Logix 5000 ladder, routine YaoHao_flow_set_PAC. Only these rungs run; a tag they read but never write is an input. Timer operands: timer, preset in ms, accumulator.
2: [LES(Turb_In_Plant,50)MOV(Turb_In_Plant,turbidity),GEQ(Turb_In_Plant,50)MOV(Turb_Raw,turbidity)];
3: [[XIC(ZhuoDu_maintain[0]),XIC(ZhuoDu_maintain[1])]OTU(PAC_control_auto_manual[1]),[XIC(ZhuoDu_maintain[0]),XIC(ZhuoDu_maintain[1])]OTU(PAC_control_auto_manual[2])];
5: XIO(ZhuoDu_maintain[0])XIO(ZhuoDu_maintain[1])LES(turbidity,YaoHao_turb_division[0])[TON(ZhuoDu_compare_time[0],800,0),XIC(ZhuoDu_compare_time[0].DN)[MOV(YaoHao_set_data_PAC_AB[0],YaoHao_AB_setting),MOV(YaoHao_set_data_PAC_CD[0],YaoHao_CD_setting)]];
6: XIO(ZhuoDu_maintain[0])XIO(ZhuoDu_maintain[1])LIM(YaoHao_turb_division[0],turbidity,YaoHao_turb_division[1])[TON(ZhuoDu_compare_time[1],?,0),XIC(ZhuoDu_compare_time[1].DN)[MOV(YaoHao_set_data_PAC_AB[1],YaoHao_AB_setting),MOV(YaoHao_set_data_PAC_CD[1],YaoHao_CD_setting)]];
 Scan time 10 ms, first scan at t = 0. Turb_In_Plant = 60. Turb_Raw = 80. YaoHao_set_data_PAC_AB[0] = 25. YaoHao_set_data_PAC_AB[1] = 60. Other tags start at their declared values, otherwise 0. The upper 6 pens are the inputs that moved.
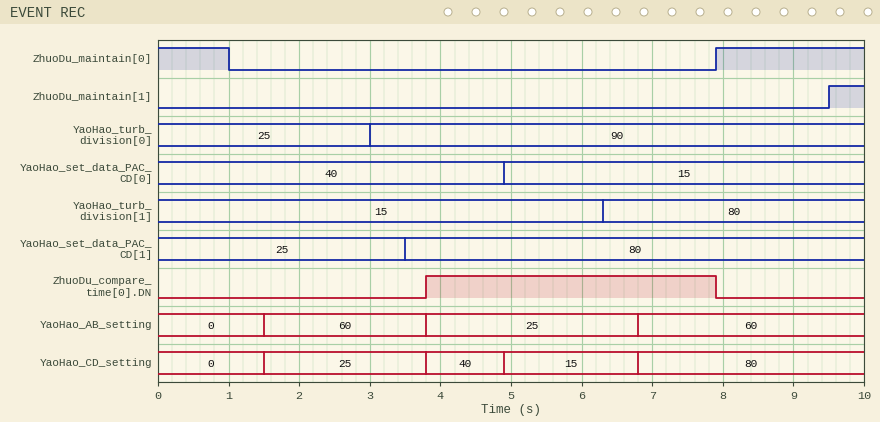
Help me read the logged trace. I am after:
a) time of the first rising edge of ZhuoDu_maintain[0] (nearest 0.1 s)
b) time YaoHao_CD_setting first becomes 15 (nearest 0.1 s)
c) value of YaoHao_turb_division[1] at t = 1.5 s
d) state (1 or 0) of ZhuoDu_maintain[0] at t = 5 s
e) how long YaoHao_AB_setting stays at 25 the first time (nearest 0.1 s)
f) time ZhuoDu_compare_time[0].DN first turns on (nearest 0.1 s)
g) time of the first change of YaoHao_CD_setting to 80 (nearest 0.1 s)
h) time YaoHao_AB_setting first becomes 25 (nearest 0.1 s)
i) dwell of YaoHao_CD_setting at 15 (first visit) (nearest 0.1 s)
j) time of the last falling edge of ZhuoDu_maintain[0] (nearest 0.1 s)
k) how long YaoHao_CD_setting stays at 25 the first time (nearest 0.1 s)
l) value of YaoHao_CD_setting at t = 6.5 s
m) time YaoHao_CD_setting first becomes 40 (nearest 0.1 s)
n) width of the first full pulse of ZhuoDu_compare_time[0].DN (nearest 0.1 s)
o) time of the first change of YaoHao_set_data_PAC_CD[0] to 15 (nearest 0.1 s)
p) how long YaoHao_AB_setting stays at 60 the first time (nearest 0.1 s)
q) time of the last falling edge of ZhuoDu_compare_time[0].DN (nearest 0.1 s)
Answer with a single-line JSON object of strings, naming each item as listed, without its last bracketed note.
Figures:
{"time of the first rising edge of ZhuoDu_maintain[0]": "7.9 s", "time YaoHao_CD_setting first becomes 15": "4.9 s", "value of YaoHao_turb_division[1] at t = 1.5 s": "15", "state (1 or 0) of ZhuoDu_maintain[0] at t = 5 s": "0", "how long YaoHao_AB_setting stays at 25 the first time": "3.0 s", "time ZhuoDu_compare_time[0].DN first turns on": "3.8 s", "time of the first change of YaoHao_CD_setting to 80": "6.8 s", "time YaoHao_AB_setting first becomes 25": "3.8 s", "dwell of YaoHao_CD_setting at 15 (first visit)": "1.9 s", "time of the last falling edge of ZhuoDu_maintain[0]": "1.0 s", "how long YaoHao_CD_setting stays at 25 the first time": "2.3 s", "value of YaoHao_CD_setting at t = 6.5 s": "15", "time YaoHao_CD_setting first becomes 40": "3.8 s", "width of the first full pulse of ZhuoDu_compare_time[0].DN": "4.1 s", "time of the first change of YaoHao_set_data_PAC_CD[0] to 15": "4.9 s", "how long YaoHao_AB_setting stays at 60 the first time": "2.3 s", "time of the last falling edge of ZhuoDu_compare_time[0].DN": "7.9 s"}
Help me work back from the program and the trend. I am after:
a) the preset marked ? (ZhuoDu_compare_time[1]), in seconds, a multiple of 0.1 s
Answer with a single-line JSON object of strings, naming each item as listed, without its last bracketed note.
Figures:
{"the preset marked ? (ZhuoDu_compare_time[1]), in seconds, a multiple of 0.1 s": "0.5 s"}
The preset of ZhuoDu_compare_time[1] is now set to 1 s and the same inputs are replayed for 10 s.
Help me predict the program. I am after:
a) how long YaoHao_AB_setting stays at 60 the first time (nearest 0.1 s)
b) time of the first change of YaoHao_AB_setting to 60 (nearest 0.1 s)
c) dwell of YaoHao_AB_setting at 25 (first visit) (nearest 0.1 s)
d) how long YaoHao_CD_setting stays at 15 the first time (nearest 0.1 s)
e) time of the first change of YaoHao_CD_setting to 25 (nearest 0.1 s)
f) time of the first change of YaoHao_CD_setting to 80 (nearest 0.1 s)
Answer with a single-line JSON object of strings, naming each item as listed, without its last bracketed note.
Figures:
{"how long YaoHao_AB_setting stays at 60 the first time": "1.8 s", "time of the first change of YaoHao_AB_setting to 60": "2.0 s", "dwell of YaoHao_AB_setting at 25 (first visit)": "3.5 s", "how long YaoHao_CD_setting stays at 15 the first time": "2.4 s", "time of the first change of YaoHao_CD_setting to 25": "2.0 s", "time of the first change of YaoHao_CD_setting to 80": "7.3 s"}
